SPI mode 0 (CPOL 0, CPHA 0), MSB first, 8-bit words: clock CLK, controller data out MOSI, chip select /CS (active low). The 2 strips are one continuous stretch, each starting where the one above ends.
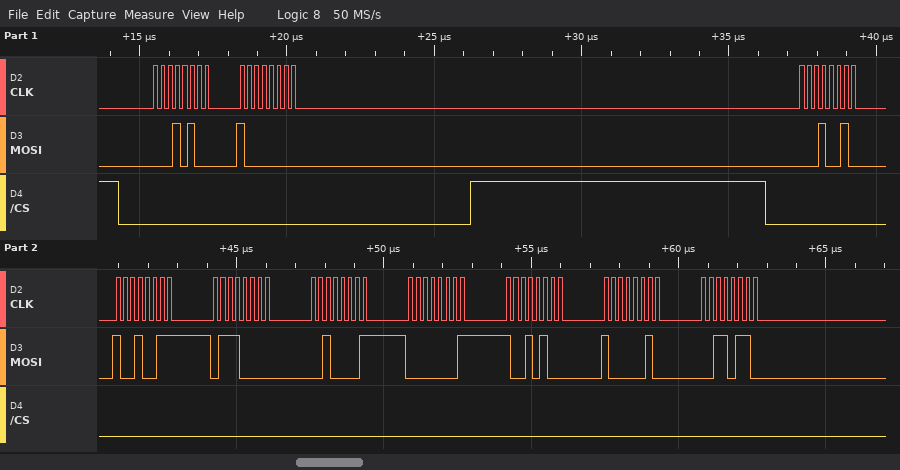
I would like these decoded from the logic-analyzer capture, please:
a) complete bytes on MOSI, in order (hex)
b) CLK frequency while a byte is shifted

14 80 12 93 70 21 01 94 82 36
4 MHz
